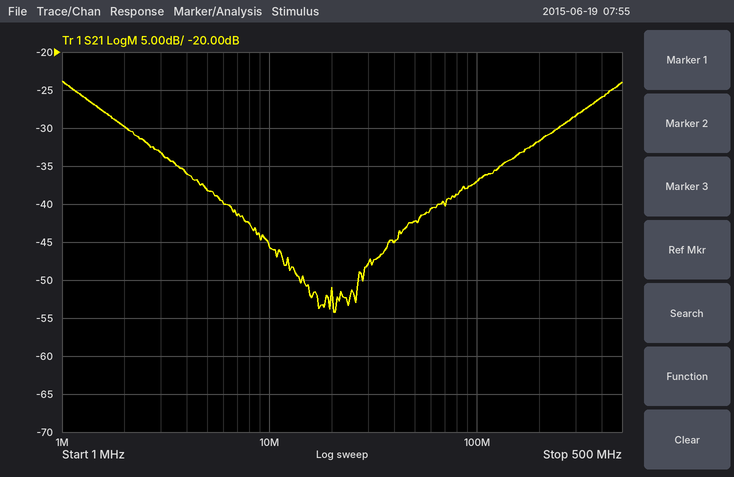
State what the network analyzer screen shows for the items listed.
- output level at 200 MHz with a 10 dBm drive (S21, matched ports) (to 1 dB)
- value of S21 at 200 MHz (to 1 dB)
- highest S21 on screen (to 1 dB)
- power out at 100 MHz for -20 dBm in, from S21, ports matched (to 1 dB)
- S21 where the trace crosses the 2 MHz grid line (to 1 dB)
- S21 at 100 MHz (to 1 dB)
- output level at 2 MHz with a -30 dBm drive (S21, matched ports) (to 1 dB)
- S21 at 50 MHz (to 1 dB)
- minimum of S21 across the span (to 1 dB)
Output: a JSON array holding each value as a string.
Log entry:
["-22 dBm", "-32 dB", "-24 dB", "-57 dBm", "-30 dB", "-37 dB", "-60 dBm", "-42 dB", "-54 dB"]
